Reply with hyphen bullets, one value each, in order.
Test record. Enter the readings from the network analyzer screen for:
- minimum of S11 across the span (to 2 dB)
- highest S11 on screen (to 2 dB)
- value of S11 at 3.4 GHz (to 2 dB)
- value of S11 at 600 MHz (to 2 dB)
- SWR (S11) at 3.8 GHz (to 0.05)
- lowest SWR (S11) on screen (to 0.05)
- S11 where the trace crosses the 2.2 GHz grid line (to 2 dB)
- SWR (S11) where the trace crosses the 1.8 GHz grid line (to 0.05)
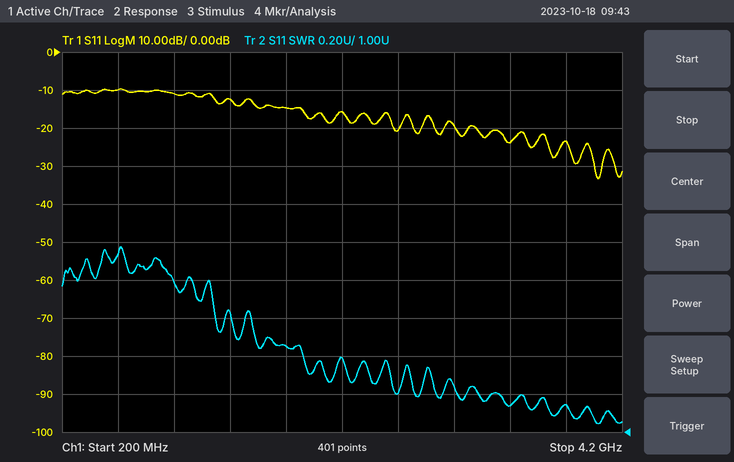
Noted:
- -34 dB
- -10 dB
- -24 dB
- -10 dB
- 1.15
- 1.05
- -16 dB
- 1.45
